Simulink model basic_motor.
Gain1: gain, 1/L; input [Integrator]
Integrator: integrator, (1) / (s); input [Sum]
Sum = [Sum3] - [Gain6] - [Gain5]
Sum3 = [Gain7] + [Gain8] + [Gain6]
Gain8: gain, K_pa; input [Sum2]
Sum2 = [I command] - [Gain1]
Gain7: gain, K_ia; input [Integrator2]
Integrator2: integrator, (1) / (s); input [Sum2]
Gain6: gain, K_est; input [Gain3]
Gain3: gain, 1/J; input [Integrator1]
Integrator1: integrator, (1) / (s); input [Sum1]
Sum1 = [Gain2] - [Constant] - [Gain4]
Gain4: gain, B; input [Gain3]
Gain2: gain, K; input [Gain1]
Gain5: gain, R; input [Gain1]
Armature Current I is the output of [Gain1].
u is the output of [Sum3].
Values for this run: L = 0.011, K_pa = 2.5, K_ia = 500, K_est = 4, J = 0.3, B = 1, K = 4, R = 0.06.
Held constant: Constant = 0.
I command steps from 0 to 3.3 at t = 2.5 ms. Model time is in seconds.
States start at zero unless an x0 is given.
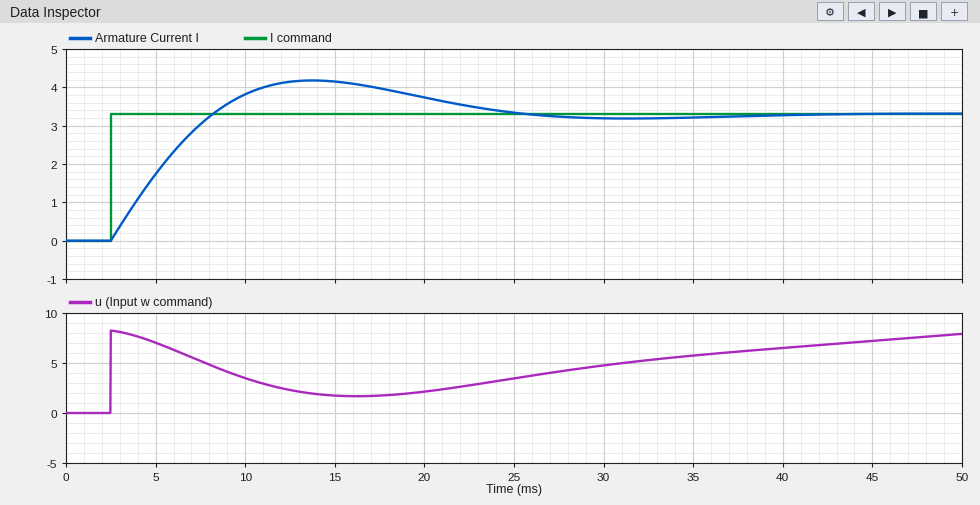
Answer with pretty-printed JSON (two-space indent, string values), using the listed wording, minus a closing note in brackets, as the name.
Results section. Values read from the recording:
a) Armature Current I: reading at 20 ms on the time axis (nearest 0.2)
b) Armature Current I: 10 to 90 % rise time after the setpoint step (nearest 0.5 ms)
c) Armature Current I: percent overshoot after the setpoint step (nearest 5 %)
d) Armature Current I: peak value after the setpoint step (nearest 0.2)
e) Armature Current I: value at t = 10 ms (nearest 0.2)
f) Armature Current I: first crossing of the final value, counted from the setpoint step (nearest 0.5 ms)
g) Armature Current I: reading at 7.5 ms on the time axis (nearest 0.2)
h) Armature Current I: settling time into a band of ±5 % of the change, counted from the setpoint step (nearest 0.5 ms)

{
  "Armature Current I: reading at 20 ms on the time axis": "3.8",
  "Armature Current I: 10 to 90 % rise time after the setpoint step": "4.5 ms",
  "Armature Current I: percent overshoot after the setpoint step": "25 %",
  "Armature Current I: peak value after the setpoint step": "4.2",
  "Armature Current I: value at t = 10 ms": "3.8",
  "Armature Current I: first crossing of the final value, counted from the setpoint step": "5.5 ms",
  "Armature Current I: reading at 7.5 ms on the time axis": "3.0",
  "Armature Current I: settling time into a band of ±5 % of the change, counted from the setpoint step": "20.5 ms"
}
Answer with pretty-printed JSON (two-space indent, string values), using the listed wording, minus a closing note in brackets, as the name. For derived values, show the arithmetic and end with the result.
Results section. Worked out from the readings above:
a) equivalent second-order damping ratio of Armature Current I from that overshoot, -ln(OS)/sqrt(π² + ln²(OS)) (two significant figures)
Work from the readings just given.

{
  "equivalent second-order damping ratio of Armature Current I from that overshoot, -ln(OS)/sqrt(π² + ln²(OS))": "ln(0.25) = -1.386; 1.386 / sqrt(9.870 + 1.922) = 0.40"
}
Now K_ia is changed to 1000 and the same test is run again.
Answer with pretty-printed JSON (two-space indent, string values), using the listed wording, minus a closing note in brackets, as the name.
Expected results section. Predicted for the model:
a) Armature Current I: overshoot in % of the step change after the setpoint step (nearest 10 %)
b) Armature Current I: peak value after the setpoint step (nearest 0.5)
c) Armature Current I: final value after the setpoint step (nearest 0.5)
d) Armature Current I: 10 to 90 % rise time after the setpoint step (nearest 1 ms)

{
  "Armature Current I: overshoot in % of the step change after the setpoint step": "40 %",
  "Armature Current I: peak value after the setpoint step": "4.5",
  "Armature Current I: final value after the setpoint step": "3.5",
  "Armature Current I: 10 to 90 % rise time after the setpoint step": "3 ms"
}
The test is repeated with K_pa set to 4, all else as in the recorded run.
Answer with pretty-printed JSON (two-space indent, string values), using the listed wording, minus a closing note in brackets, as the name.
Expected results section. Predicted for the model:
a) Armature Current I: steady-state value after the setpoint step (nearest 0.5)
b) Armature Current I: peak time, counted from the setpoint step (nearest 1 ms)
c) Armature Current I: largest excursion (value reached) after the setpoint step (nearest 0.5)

{
  "Armature Current I: steady-state value after the setpoint step": "3.5",
  "Armature Current I: peak time, counted from the setpoint step": "10 ms",
  "Armature Current I: largest excursion (value reached) after the setpoint step": "4.0"
}
